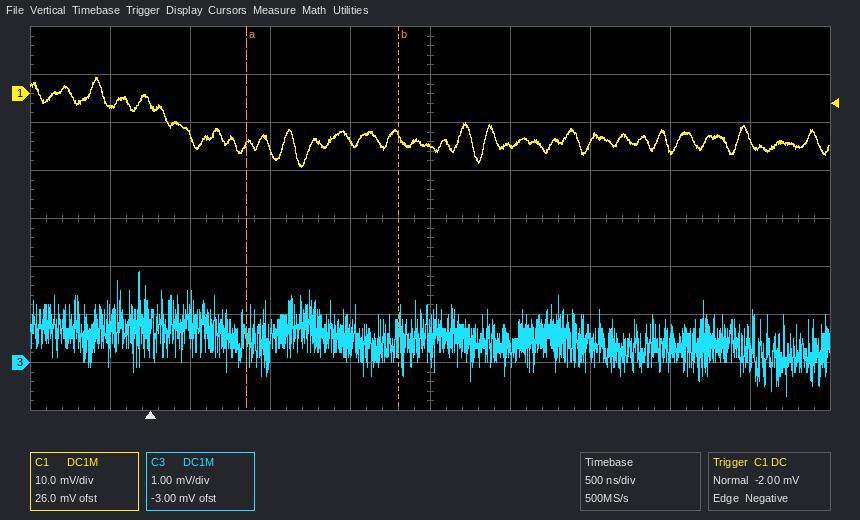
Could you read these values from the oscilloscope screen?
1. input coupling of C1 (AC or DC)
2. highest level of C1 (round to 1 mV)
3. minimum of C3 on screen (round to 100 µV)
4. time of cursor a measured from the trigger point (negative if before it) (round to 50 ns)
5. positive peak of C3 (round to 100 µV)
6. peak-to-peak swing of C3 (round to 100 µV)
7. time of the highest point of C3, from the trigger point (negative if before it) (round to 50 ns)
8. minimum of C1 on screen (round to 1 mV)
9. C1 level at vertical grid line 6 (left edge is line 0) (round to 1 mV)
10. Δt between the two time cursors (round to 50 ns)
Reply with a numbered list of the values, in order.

1. DC
2. 3 mV
3. -700 µV
4. +600 ns
5. 1.9 mV
6. 2.6 mV
7. -50 ns
8. -15 mV
9. -11 mV
10. 950 ns
